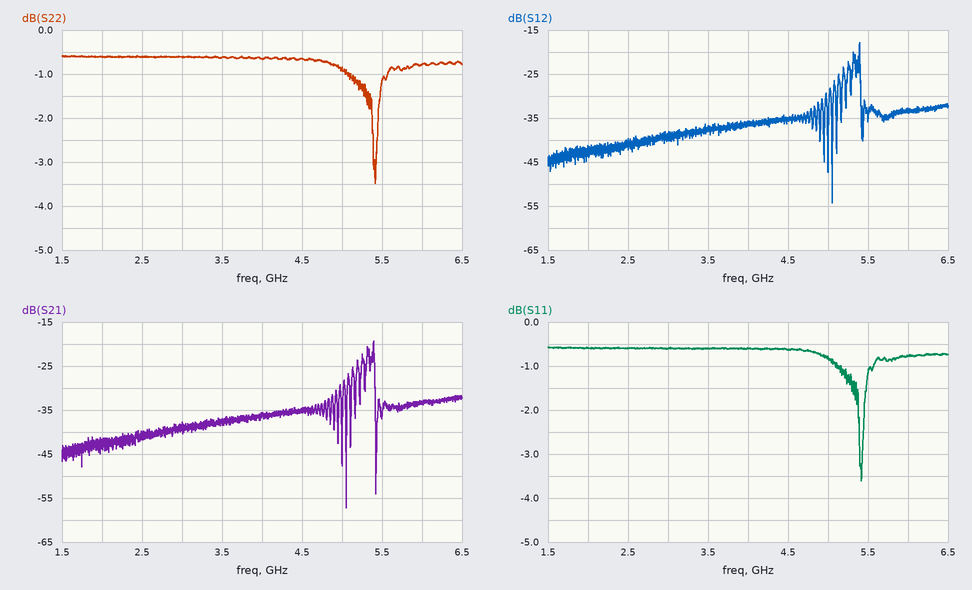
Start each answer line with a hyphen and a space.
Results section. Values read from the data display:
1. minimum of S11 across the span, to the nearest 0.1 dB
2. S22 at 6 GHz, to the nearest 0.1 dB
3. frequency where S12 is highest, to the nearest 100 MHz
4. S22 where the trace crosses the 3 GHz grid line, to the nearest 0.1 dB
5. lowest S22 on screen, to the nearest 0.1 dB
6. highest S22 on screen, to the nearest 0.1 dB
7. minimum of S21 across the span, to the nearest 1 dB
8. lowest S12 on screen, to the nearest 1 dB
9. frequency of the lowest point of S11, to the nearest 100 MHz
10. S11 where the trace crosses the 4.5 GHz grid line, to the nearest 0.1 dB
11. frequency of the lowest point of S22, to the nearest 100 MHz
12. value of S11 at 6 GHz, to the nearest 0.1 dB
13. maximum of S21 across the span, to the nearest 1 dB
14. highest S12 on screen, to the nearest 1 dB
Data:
- -3.6 dB
- -0.8 dB
- 5.4 GHz
- -0.6 dB
- -3.5 dB
- -0.6 dB
- -57 dB
- -54 dB
- 5.4 GHz
- -0.6 dB
- 5.4 GHz
- -0.8 dB
- -19 dB
- -18 dB
